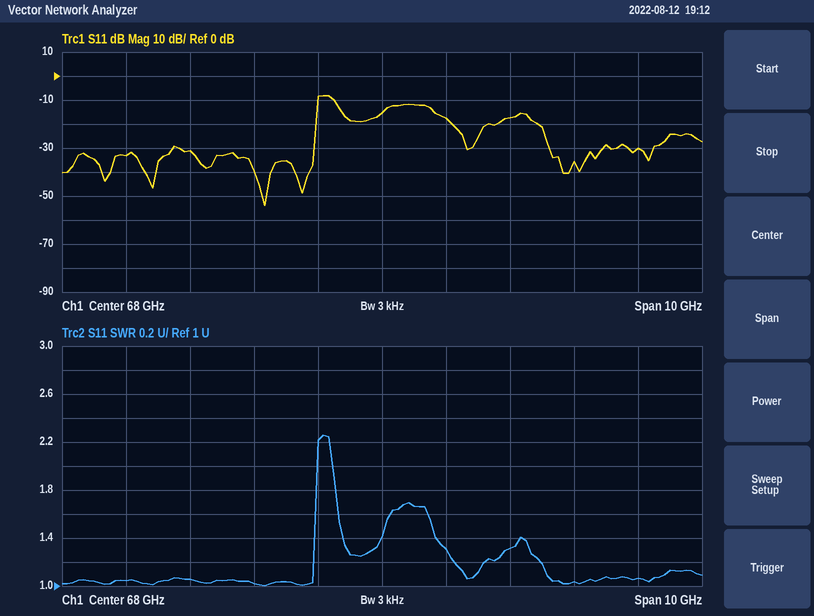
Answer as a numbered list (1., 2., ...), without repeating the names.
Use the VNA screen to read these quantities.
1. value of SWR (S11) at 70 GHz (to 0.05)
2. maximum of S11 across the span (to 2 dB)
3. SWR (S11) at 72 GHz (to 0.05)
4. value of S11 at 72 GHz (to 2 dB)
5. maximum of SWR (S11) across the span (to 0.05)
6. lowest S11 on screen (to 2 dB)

1. 1.30
2. -8 dB
3. 1.05
4. -30 dB
5. 2.25
6. -54 dB
